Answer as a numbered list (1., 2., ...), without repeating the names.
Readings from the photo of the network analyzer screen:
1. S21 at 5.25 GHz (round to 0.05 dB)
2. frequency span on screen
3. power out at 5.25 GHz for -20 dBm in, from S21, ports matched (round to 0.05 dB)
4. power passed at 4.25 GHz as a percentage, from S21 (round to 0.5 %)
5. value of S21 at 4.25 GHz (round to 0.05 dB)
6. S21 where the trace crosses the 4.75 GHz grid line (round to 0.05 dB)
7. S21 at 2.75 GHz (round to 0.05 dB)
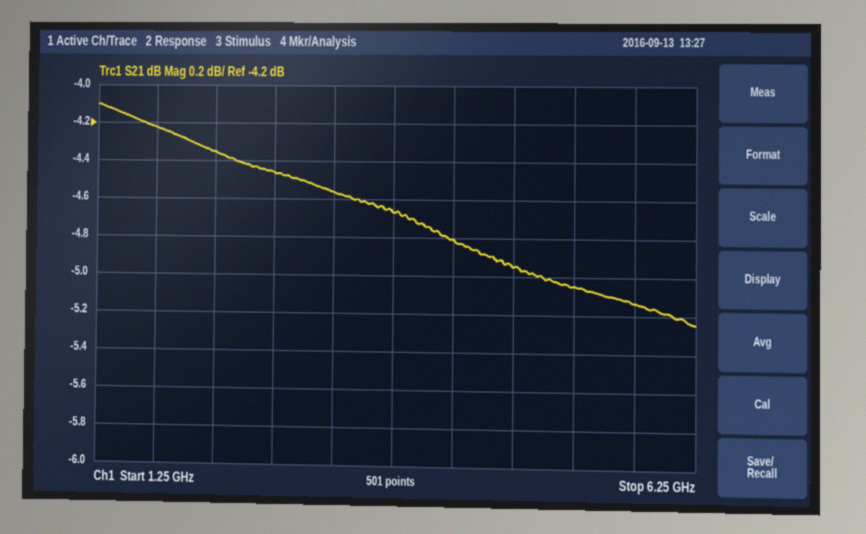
1. -5.05 dB
2. 5 GHz
3. -25.05 dBm
4. 33.0 %
5. -4.80 dB
6. -4.95 dB
7. -4.45 dB
